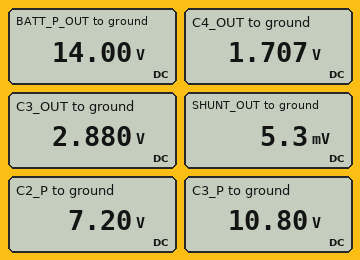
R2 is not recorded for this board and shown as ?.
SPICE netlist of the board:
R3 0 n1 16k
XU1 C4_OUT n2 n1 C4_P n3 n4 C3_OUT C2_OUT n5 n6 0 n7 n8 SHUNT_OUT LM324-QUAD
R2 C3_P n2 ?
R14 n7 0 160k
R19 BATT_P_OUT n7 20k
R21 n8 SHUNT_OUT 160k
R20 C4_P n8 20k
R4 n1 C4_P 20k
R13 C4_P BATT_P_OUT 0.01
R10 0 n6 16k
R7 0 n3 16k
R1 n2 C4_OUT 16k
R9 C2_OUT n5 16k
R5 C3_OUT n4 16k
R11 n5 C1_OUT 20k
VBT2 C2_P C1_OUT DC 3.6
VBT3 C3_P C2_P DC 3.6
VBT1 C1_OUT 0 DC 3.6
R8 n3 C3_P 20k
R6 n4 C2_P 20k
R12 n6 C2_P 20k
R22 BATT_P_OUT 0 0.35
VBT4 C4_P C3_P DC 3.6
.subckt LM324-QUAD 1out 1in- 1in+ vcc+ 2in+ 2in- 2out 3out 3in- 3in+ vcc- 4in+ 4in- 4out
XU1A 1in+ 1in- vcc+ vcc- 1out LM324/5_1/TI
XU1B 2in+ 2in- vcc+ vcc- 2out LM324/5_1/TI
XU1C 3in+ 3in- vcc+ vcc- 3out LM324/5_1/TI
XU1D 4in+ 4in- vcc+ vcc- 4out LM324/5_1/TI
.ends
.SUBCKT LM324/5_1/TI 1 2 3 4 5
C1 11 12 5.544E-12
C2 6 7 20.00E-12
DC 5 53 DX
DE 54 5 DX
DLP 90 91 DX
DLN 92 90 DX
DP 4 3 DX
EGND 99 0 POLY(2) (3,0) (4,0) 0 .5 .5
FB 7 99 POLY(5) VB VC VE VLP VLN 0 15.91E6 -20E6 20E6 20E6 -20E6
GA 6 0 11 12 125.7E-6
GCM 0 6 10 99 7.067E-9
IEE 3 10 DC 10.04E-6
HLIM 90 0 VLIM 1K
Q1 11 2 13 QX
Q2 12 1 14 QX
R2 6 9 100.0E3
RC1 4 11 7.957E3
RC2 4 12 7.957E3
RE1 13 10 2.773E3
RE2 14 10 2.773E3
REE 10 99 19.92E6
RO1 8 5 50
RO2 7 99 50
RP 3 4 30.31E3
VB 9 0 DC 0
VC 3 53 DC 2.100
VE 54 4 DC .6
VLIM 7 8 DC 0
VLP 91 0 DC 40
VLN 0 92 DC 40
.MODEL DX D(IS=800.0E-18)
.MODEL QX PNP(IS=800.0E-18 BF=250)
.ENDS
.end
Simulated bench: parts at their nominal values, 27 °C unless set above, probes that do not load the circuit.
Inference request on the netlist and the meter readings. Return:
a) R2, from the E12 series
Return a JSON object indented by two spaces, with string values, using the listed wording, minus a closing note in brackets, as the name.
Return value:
{
  "R2, from the E12 series": "15 kΩ"
}
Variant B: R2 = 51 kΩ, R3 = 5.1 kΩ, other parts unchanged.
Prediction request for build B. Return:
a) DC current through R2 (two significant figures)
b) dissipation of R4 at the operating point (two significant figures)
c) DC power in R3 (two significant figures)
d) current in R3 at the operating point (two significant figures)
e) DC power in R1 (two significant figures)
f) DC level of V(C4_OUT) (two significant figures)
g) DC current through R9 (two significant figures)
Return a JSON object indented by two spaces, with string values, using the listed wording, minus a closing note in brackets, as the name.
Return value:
{
  "DC current through R2": "150 µA",
  "dissipation of R4 at the operating point": "6.6 mW",
  "DC power in R3": "1.7 mW",
  "current in R3 at the operating point": "570 µA",
  "DC power in R1": "380 µW",
  "DC level of V(C4_OUT)": "460 mV",
  "DC current through R9": "20 µA"
}
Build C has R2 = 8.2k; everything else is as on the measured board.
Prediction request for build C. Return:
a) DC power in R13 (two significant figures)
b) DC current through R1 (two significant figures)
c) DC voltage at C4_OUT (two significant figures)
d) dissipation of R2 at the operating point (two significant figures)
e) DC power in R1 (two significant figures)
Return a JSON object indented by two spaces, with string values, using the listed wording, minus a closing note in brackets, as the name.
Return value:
{
  "DC power in R13": "16 W",
  "DC current through R1": "450 µA",
  "DC voltage at C4_OUT": "4.6 mV",
  "dissipation of R2 at the operating point": "1.6 mW",
  "DC power in R1": "3.2 mW"
}
